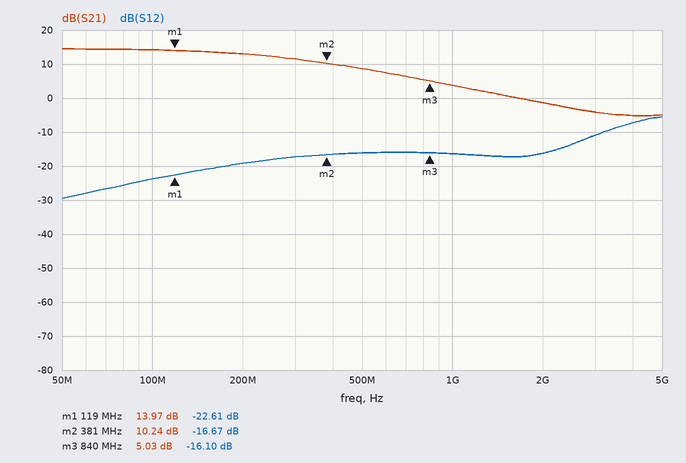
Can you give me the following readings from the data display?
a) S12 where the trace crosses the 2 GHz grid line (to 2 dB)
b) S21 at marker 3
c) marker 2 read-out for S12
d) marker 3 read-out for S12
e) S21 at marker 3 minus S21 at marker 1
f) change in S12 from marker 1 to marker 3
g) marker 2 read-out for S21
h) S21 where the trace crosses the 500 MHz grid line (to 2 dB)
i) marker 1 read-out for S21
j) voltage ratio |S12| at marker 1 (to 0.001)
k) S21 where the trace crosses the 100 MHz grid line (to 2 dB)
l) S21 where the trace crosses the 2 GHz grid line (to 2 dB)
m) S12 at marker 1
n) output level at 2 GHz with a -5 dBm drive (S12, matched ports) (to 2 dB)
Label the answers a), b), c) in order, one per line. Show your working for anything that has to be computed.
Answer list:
a) -16 dB
b) 5.03 dB
c) -16.67 dB
d) -16.10 dB
e) 5.03 − (13.97) = -8.94 dB
f) -16.1 − (-22.61) = 6.51 dB
g) 10.24 dB
h) 8 dB
i) 13.97 dB
j) 10^(-22.61/20) ≈ 0.074
k) 14 dB
l) -2 dB
m) -22.61 dB
n) -5 dBm + (-16 dB) = -22 dBm
